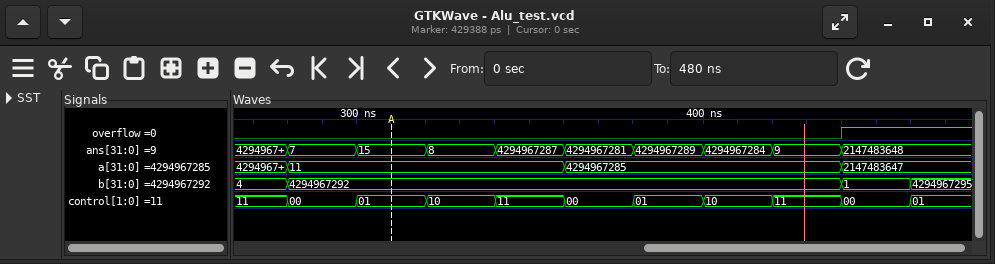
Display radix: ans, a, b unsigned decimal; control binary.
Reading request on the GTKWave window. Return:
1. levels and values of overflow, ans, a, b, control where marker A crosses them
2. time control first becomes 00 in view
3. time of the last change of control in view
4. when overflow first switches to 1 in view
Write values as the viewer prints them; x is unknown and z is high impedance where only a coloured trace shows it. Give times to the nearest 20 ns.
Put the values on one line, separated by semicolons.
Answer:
overflow=0, ans=15, a=11, b=4294967292, control=01; 280 ns; 460 ns; 440 ns
